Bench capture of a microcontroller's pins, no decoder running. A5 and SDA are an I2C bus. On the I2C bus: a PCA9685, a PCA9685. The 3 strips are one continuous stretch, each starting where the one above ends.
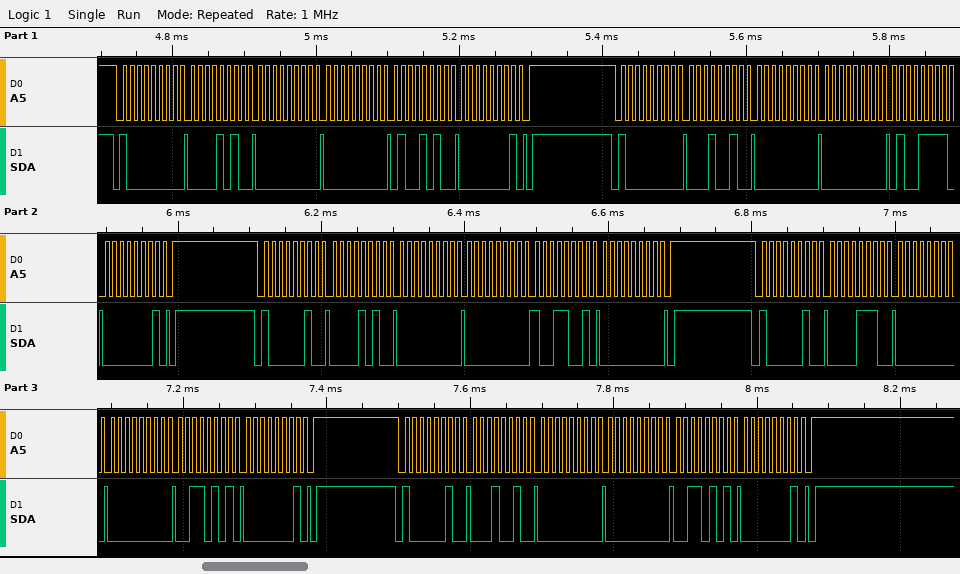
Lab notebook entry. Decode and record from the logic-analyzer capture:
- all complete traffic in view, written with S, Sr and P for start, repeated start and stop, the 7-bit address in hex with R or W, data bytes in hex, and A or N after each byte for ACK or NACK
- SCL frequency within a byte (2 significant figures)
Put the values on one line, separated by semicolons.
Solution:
S 40W A 0A A 00 A 00 A 4A A 01 A P S 40W A 12 A 00 A 00 A 4F A 01 A P S 41W A 0A A 00 A 00 A 99 A 00 A P S 41W A 0E A 00 A 00 A 35 A 01 A P S 41W A 12 A 00 A 00 A 35 A 01 A P; 100 kHz
